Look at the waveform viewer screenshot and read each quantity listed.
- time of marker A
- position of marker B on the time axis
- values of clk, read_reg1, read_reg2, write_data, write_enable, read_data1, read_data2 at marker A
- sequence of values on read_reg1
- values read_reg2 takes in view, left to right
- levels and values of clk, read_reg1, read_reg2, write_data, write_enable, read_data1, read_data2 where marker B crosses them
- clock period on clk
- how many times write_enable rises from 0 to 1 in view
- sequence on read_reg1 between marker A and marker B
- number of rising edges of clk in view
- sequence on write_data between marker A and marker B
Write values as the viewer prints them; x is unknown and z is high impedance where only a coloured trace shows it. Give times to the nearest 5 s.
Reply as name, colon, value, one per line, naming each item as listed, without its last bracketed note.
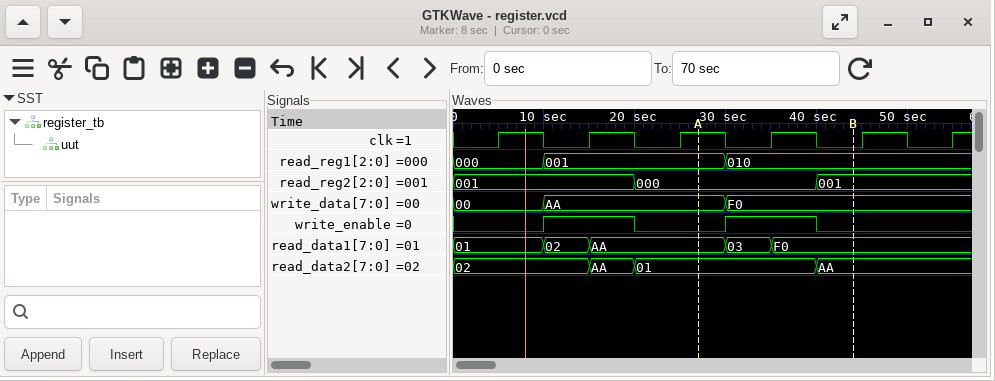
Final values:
time of marker A: 25 s
position of marker B on the time axis: 45 s
values of clk, read_reg1, read_reg2, write_data, write_enable, read_data1, read_data2 at marker A: clk=1, read_reg1=001, read_reg2=000, write_data=AA, write_enable=0, read_data1=AA, read_data2=01
sequence of values on read_reg1: 000, 001, 010
values read_reg2 takes in view, left to right: 001, 000, 001
levels and values of clk, read_reg1, read_reg2, write_data, write_enable, read_data1, read_data2 where marker B crosses them: clk=0, read_reg1=010, read_reg2=001, write_data=F0, write_enable=0, read_data1=F0, read_data2=AA
clock period on clk: 10 s
how many times write_enable rises from 0 to 1 in view: 2
sequence on read_reg1 between marker A and marker B: 001, 010
number of rising edges of clk in view: 6
sequence on write_data between marker A and marker B: AA, F0
